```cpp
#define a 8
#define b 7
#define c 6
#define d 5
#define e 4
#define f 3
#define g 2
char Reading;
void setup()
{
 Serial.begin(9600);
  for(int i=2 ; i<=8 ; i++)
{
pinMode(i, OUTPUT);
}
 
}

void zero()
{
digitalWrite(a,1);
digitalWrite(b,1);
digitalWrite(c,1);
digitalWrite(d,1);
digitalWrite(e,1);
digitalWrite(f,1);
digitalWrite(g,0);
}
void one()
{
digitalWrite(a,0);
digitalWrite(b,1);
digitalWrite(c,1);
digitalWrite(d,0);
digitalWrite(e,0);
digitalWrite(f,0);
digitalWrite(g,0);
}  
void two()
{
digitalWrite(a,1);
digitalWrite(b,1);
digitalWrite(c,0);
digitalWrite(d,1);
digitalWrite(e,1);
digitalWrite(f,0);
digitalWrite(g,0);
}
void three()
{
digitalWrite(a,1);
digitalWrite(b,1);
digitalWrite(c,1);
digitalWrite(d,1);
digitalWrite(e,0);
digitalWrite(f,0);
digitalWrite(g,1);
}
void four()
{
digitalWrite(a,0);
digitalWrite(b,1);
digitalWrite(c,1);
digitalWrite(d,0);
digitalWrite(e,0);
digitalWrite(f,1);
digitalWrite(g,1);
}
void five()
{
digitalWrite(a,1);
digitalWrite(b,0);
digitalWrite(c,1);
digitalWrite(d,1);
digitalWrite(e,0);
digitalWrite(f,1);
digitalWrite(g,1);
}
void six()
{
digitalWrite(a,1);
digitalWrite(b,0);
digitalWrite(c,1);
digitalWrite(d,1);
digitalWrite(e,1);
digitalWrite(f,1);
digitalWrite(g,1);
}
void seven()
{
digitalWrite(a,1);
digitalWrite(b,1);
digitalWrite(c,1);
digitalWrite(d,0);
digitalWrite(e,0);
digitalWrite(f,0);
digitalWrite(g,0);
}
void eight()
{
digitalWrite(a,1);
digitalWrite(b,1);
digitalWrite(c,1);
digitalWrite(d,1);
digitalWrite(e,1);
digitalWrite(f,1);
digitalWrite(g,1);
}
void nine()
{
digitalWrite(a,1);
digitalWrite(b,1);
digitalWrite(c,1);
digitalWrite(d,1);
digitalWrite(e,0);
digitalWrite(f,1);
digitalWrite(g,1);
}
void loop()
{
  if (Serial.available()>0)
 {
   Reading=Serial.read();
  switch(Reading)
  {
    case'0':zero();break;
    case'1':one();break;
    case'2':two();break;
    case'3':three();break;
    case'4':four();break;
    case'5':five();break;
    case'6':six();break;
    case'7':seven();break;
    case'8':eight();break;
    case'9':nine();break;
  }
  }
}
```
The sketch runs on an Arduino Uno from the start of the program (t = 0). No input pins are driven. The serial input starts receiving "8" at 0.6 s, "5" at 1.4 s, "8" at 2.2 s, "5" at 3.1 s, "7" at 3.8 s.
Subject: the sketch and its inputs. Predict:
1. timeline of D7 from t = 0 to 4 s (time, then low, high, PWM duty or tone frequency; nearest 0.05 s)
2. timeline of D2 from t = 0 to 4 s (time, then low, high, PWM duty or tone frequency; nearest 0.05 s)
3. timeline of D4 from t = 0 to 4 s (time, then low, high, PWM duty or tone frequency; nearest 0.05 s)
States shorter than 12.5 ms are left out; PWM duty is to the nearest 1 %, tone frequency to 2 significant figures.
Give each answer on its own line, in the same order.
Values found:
0 s low; 0.6 s high; 1.4 s low; 2.2 s high; 3.1 s low; 3.8 s high
0 s low; 0.6 s high; 3.8 s low
0 s low; 0.6 s high; 1.4 s low; 2.2 s high; 3.1 s low
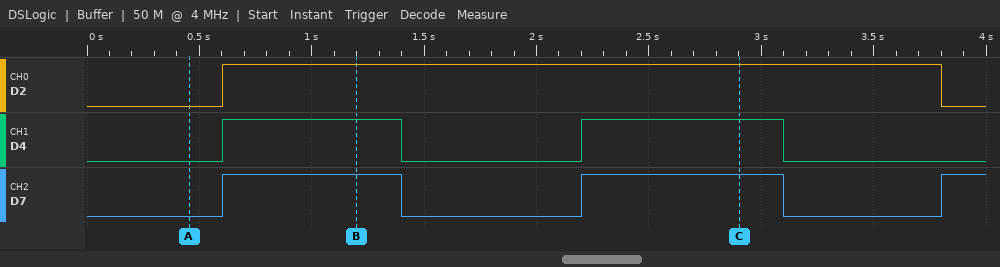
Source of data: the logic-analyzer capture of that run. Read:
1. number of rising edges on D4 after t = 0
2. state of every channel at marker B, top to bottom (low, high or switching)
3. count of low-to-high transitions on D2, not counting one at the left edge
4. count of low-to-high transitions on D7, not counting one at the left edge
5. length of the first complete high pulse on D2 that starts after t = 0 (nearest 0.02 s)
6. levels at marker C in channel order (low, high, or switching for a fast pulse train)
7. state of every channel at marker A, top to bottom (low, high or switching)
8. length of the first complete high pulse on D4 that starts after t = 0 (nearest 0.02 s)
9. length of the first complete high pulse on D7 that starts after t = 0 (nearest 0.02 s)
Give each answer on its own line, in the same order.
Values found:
2
D2 high, D4 high, D7 high
1
3
3.20 s
D2 high, D4 high, D7 high
D2 low, D4 low, D7 low
0.80 s
0.80 s
